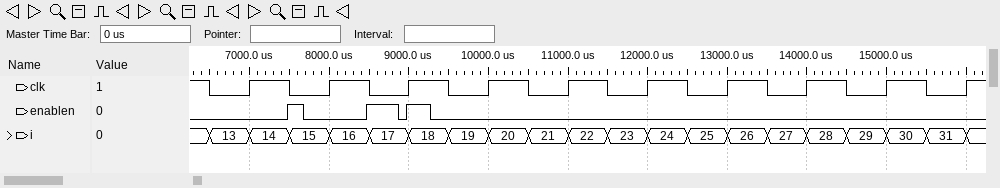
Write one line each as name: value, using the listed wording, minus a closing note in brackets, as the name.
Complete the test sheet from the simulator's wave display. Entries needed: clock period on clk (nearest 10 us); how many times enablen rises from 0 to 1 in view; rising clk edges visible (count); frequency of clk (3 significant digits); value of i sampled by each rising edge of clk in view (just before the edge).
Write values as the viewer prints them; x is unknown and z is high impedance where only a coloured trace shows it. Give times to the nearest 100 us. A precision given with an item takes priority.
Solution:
clock period on clk: 1000 us
how many times enablen rises from 0 to 1 in view: 3
rising clk edges visible: 10
frequency of clk: 1.00 kHz
value of i sampled by each rising edge of clk in view: 13, 15, 17, 19, 21, 23, 25, 27, 29, 31
